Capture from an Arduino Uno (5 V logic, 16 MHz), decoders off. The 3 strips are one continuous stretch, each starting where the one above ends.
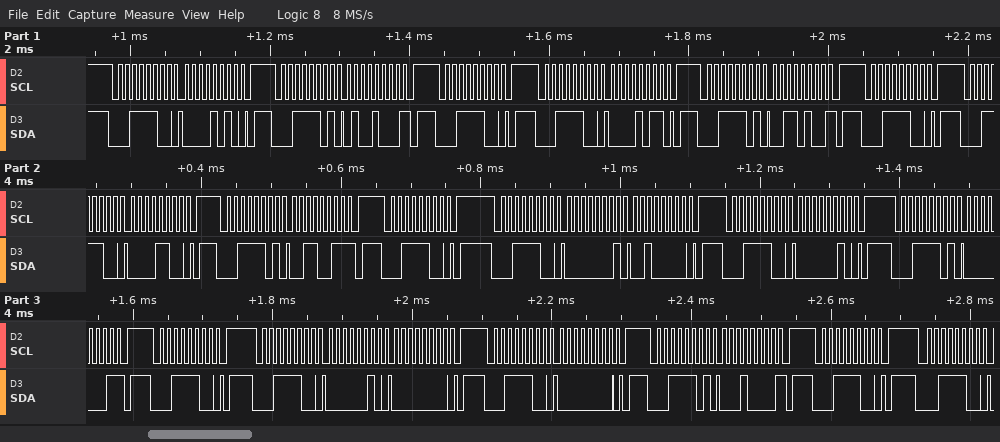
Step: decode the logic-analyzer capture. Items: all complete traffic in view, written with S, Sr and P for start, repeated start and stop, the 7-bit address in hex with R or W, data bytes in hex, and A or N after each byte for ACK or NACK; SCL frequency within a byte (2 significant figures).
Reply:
S 1EW A 0A A P S 1ER A 48 N P S 1EW A P S 1EW A 0B A P S 1ER A 34 N P S 1EW A P S 1EW A 0C A P S 1ER A 33 N P S 1EW A P S 1EW A 01 A 20 A P S 1EW A 02 A P S 1ER A 01 N P S 1EW A P S 1EW A 02 A 00 A P S 1EW A 00 A P S 1ER A 10 N P S 1EW A P S 1EW A
100 kHz
